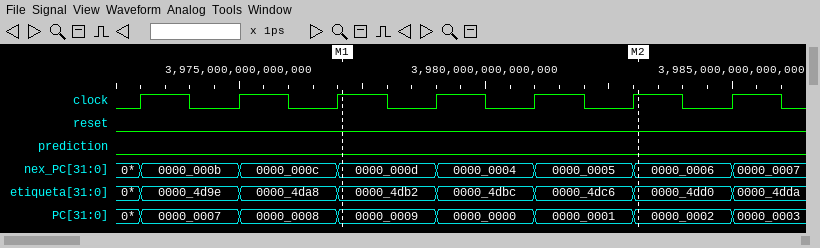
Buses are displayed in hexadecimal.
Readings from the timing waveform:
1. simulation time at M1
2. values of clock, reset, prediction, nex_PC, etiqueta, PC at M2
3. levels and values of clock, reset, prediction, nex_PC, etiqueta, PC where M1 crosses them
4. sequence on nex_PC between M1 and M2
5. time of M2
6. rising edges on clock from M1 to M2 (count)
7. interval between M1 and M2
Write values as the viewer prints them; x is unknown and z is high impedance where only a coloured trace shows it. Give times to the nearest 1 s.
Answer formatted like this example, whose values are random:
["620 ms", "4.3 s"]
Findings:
["3977 s", "clock=1, reset=0, prediction=0, nex_PC=0000_0006, etiqueta=0000_4dd0, PC=0000_0002", "clock=1, reset=0, prediction=0, nex_PC=0000_000d, etiqueta=0000_4db2, PC=0000_0009", "0000_000d, 0000_0004, 0000_0005, 0000_0006", "3983 s", "3", "6 s"]
